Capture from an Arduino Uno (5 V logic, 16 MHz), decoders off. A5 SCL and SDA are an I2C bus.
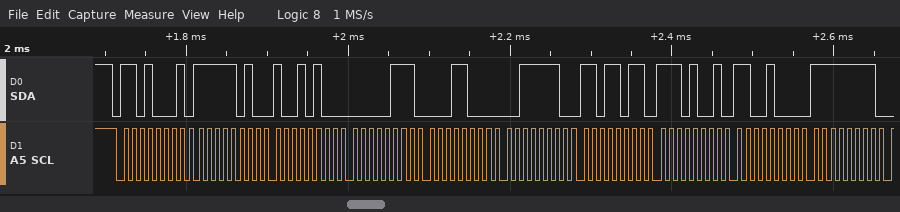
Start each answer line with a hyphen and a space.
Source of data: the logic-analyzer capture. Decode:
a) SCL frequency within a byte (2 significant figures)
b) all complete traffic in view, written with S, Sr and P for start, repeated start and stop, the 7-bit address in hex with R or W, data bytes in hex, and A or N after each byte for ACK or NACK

- 100 kHz
- S 68R A FA A 94 A 07 A 18 A 3E A DB A E9 A C8 A FF A
